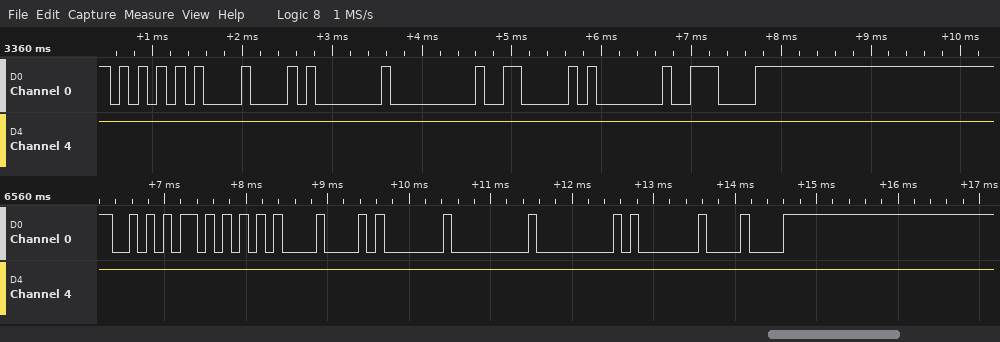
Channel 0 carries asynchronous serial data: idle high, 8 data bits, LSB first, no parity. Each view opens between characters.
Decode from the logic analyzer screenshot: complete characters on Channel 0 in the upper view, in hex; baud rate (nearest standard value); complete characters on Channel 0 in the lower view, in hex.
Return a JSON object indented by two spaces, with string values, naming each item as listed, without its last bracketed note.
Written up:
{
  "complete characters on Channel 0 in the upper view, in hex": "55, 08, 01, 00, 06, 01, 0E",
  "baud rate": "9600 baud",
  "complete characters on Channel 0 in the lower view, in hex": "AA, 55, 08, 01, 00, 00, 01, 08"
}
